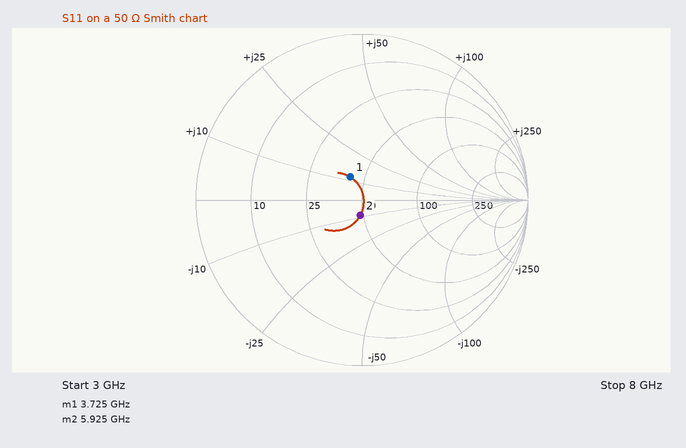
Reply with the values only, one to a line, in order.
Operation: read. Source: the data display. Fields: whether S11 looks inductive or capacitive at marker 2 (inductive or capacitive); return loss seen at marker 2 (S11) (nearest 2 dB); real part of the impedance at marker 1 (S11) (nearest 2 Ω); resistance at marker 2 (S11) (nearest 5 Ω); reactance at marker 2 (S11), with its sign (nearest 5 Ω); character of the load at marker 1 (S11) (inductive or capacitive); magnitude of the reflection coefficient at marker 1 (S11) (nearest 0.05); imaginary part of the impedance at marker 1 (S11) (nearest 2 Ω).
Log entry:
capacitive
20 dB
42 Ω
50 Ω
-10 Ω
inductive
0.15
+12 Ω
